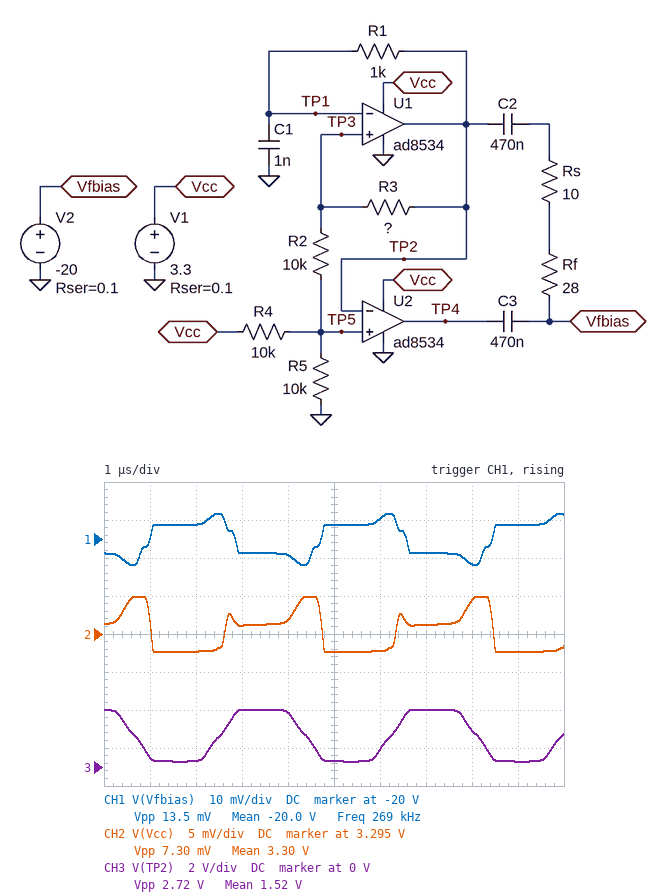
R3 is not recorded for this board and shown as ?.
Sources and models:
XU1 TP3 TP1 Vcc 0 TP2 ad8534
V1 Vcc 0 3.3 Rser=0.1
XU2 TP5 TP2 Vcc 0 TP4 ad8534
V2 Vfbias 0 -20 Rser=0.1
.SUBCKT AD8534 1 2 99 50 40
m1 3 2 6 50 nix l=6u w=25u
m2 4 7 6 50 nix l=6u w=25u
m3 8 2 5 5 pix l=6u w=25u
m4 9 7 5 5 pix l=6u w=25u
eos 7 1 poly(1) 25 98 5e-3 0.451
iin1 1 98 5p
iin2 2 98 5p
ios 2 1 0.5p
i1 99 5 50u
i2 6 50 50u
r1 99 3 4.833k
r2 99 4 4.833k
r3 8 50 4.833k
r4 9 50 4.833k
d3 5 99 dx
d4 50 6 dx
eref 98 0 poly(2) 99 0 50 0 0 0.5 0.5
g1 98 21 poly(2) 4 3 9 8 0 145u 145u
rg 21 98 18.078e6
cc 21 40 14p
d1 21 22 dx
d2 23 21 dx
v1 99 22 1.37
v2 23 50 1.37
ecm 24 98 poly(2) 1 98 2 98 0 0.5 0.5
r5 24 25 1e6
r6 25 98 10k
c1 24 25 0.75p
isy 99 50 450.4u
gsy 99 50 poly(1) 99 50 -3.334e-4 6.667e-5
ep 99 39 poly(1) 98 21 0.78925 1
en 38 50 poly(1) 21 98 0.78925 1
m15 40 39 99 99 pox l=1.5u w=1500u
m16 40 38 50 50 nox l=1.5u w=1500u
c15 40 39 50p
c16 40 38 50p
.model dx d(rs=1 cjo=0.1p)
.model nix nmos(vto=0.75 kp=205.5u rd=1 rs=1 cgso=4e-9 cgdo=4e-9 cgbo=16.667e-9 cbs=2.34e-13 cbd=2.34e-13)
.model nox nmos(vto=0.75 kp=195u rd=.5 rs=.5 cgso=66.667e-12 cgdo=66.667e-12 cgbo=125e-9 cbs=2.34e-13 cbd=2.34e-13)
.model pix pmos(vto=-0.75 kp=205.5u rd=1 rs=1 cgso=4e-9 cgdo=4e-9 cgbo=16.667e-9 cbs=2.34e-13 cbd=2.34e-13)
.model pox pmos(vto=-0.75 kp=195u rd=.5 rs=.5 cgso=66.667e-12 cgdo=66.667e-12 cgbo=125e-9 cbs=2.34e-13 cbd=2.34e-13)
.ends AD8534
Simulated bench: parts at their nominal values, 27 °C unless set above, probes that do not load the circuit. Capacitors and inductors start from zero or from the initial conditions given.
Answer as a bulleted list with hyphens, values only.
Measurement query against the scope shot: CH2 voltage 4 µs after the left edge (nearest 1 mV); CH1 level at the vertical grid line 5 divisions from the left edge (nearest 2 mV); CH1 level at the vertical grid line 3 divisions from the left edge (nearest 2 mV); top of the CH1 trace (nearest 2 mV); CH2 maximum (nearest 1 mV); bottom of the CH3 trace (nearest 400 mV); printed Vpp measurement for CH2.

- 3.297 V
- -19.996 V
- -20.004 V
- -19.994 V
- 3.300 V
- 400 mV
- 7.30 mV
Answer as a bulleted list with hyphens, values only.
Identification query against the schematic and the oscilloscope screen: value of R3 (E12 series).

- 15 kΩ
